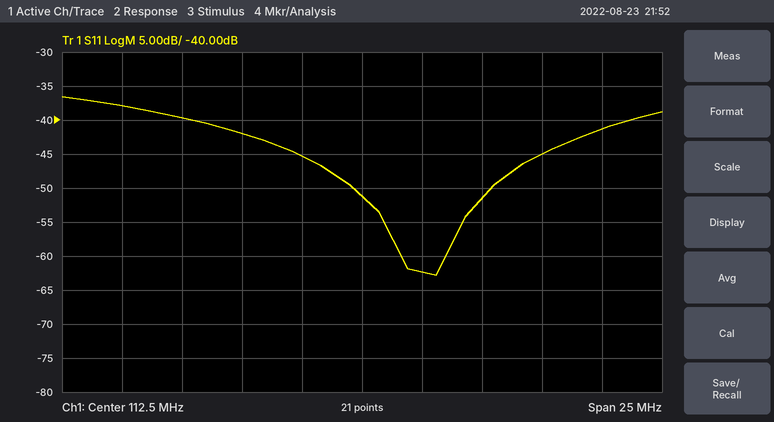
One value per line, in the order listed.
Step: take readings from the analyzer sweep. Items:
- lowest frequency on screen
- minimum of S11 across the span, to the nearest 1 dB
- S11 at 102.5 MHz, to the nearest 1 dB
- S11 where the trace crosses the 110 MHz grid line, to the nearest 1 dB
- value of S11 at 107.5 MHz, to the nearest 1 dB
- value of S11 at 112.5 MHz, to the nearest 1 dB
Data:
100 MHz
-63 dB
-38 dB
-45 dB
-42 dB
-51 dB
